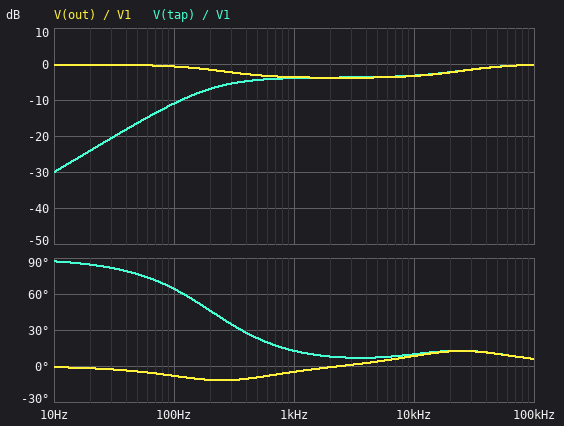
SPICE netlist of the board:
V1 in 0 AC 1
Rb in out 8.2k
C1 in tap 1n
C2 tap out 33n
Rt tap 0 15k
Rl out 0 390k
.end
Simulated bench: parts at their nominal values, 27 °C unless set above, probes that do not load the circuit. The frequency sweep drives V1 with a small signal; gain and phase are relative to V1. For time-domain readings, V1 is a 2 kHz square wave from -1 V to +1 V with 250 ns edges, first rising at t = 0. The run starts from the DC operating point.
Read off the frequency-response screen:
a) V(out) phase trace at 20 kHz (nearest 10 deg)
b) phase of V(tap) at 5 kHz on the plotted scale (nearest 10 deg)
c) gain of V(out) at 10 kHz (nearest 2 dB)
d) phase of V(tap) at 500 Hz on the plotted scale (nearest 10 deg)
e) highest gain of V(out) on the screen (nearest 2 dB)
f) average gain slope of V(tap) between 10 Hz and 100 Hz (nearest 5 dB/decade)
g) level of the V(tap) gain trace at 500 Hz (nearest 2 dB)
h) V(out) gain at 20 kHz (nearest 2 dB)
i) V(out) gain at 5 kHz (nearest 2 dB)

10 deg
10 deg
-4 dB
20 deg
0 dB
20 dB/decade
-4 dB
-2 dB
-4 dB
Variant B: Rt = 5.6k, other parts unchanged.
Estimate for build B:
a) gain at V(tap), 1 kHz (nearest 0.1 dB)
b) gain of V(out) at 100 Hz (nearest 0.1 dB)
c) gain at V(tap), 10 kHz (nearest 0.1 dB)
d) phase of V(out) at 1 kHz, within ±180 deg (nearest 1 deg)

-8.2 dB
-0.5 dB
-6.9 dB
-20 deg
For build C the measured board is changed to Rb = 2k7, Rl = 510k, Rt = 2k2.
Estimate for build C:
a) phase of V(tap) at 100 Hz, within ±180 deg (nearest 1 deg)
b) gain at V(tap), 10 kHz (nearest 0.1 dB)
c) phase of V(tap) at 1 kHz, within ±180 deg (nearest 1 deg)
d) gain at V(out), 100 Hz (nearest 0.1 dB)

84 deg
-6.7 dB
45 deg
-0.1 dB
